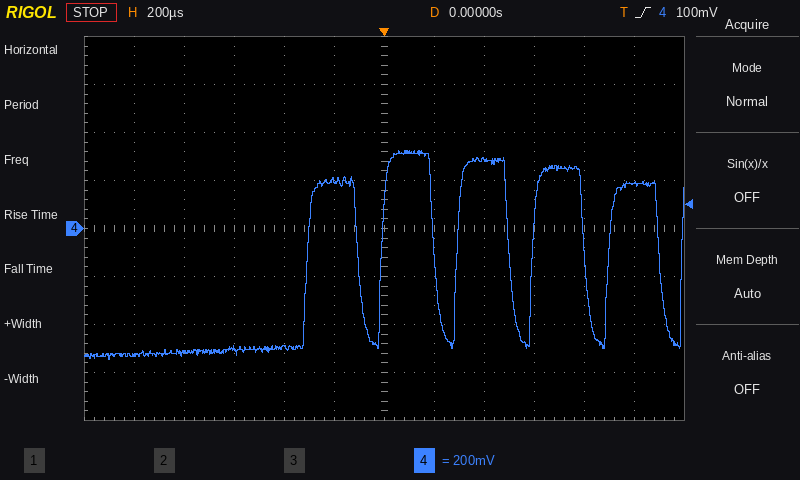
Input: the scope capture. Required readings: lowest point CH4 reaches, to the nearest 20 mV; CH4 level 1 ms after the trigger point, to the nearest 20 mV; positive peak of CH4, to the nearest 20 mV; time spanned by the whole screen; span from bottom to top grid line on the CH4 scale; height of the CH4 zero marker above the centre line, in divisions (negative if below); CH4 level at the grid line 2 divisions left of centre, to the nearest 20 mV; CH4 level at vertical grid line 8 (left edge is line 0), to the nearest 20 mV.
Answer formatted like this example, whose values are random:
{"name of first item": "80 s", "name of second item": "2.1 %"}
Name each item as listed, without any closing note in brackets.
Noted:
{"lowest point CH4 reaches, to the nearest 20 mV": "-540 mV", "CH4 level 1 ms after the trigger point, to the nearest 20 mV": "180 mV", "positive peak of CH4, to the nearest 20 mV": "320 mV", "time spanned by the whole screen": "2.4 ms", "span from bottom to top grid line on the CH4 scale": "1.6 V", "height of the CH4 zero marker above the centre line, in divisions": "0.0 div", "CH4 level at the grid line 2 divisions left of centre, to the nearest 20 mV": "-500 mV", "CH4 level at vertical grid line 8 (left edge is line 0), to the nearest 20 mV": "280 mV"}
